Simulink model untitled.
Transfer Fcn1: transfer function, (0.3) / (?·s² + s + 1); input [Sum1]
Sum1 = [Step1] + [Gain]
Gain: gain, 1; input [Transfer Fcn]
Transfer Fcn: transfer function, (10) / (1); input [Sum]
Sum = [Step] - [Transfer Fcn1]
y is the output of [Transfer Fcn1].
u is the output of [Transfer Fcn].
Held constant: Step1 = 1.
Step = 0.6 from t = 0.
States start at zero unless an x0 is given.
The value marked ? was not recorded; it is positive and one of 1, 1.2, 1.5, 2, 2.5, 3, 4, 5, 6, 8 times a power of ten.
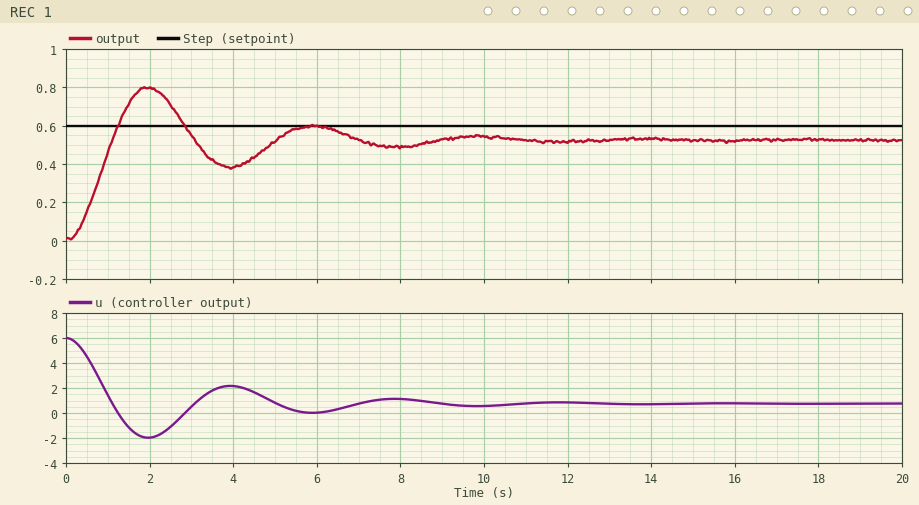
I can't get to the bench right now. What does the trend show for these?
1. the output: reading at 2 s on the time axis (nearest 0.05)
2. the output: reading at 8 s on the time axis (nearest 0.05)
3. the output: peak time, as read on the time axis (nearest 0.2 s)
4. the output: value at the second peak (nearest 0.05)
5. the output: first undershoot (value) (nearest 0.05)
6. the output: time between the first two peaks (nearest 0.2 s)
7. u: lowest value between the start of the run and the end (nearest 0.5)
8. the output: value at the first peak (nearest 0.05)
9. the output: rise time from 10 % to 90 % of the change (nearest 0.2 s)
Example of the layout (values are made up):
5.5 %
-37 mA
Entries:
0.80
0.50
2.0 s
0.60
0.40
4.0 s
-2.0
0.80
0.8 s
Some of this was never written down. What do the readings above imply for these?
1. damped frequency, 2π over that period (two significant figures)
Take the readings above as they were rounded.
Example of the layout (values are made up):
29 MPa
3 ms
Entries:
1.6 rad/s
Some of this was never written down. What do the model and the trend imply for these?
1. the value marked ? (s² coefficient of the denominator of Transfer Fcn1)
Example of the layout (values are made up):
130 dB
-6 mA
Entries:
1.5
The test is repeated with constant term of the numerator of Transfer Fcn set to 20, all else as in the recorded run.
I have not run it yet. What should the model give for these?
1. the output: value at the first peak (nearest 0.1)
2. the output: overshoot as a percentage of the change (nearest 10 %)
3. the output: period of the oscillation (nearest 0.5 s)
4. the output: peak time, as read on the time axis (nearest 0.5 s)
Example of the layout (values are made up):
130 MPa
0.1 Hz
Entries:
0.9
60 %
3.0 s
1.5 s
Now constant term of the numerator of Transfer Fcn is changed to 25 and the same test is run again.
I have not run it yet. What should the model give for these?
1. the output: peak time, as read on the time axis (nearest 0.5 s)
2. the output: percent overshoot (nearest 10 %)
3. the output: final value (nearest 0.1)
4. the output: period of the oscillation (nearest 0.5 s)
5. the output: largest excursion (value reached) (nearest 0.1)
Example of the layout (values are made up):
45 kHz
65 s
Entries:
1.5 s
60 %
0.6
2.5 s
0.9
